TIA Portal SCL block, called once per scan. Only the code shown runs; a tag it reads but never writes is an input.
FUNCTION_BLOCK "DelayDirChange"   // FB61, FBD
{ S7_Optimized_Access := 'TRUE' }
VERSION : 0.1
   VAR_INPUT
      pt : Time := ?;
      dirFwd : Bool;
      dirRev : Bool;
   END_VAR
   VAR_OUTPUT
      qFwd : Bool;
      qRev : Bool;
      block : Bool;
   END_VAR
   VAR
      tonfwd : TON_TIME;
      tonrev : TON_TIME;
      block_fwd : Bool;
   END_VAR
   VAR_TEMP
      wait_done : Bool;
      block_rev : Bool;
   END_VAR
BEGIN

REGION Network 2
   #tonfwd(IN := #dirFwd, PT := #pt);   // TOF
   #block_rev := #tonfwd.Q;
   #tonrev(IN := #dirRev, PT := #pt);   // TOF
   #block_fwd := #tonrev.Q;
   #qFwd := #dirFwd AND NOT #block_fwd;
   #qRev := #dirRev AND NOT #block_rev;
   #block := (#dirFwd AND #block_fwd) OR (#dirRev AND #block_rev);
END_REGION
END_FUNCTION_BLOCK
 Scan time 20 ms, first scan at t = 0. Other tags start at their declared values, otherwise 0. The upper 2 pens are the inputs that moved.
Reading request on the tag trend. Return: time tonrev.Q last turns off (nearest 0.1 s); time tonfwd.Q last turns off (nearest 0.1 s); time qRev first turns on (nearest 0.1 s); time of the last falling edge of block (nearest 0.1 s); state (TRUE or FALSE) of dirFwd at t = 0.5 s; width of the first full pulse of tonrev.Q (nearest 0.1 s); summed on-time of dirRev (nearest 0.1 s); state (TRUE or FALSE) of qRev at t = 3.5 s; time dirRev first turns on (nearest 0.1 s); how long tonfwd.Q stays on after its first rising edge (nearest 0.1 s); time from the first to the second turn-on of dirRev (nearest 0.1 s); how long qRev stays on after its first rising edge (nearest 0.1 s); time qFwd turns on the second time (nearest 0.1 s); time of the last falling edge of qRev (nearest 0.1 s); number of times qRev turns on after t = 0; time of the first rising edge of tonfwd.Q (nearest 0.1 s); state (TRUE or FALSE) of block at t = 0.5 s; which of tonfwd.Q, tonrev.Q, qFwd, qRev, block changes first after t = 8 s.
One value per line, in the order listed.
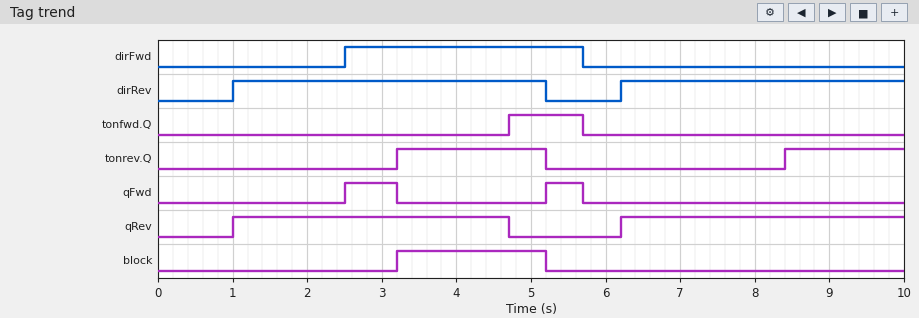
5.2 s
5.7 s
1.0 s
5.2 s
FALSE
2.0 s
8.0 s
TRUE
1.0 s
1.0 s
5.2 s
3.7 s
5.2 s
4.7 s
2
4.7 s
FALSE
tonrev.Q
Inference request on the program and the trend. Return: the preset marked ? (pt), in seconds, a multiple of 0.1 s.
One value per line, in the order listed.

2.2 s
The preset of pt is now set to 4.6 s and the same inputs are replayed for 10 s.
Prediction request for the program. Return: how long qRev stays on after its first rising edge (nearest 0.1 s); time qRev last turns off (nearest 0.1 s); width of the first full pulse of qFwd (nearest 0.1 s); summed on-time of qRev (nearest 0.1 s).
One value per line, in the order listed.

4.2 s
5.2 s
3.2 s
8.0 s
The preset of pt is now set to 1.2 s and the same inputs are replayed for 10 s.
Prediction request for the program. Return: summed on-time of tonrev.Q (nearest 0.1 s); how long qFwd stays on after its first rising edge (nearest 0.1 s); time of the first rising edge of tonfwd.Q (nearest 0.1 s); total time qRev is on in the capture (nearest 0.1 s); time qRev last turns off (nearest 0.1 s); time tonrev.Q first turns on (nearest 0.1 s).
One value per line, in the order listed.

5.6 s
0.5 s
3.7 s
6.5 s
3.7 s
2.2 s
